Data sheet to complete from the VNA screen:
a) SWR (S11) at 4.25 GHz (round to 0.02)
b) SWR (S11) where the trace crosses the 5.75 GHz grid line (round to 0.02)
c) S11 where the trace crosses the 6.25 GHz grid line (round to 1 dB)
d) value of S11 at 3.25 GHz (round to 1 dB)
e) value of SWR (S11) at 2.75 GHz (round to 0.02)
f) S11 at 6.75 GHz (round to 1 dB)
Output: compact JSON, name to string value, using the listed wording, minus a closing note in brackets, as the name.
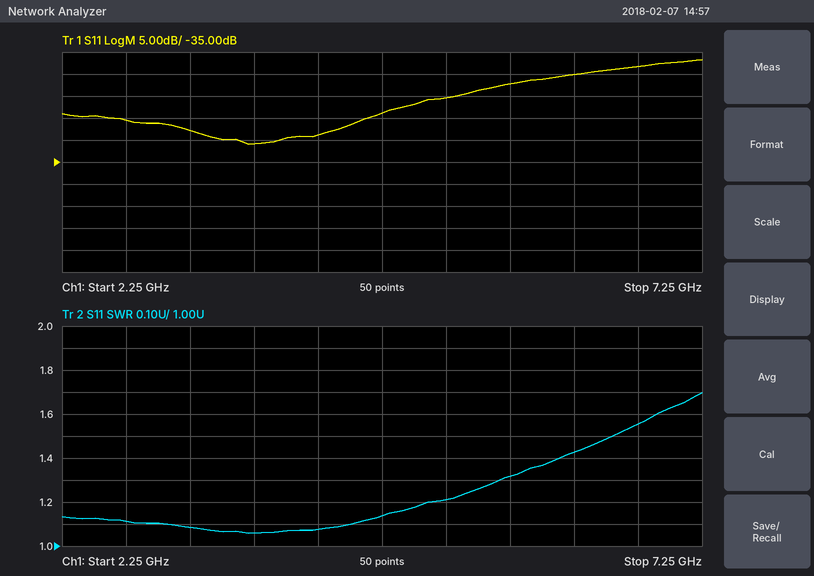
{"SWR (S11) at 4.25 GHz": "1.08", "SWR (S11) where the trace crosses the 5.75 GHz grid line": "1.32", "S11 where the trace crosses the 6.25 GHz grid line": "-15 dB", "value of S11 at 3.25 GHz": "-28 dB", "value of SWR (S11) at 2.75 GHz": "1.12", "S11 at 6.75 GHz": "-13 dB"}
